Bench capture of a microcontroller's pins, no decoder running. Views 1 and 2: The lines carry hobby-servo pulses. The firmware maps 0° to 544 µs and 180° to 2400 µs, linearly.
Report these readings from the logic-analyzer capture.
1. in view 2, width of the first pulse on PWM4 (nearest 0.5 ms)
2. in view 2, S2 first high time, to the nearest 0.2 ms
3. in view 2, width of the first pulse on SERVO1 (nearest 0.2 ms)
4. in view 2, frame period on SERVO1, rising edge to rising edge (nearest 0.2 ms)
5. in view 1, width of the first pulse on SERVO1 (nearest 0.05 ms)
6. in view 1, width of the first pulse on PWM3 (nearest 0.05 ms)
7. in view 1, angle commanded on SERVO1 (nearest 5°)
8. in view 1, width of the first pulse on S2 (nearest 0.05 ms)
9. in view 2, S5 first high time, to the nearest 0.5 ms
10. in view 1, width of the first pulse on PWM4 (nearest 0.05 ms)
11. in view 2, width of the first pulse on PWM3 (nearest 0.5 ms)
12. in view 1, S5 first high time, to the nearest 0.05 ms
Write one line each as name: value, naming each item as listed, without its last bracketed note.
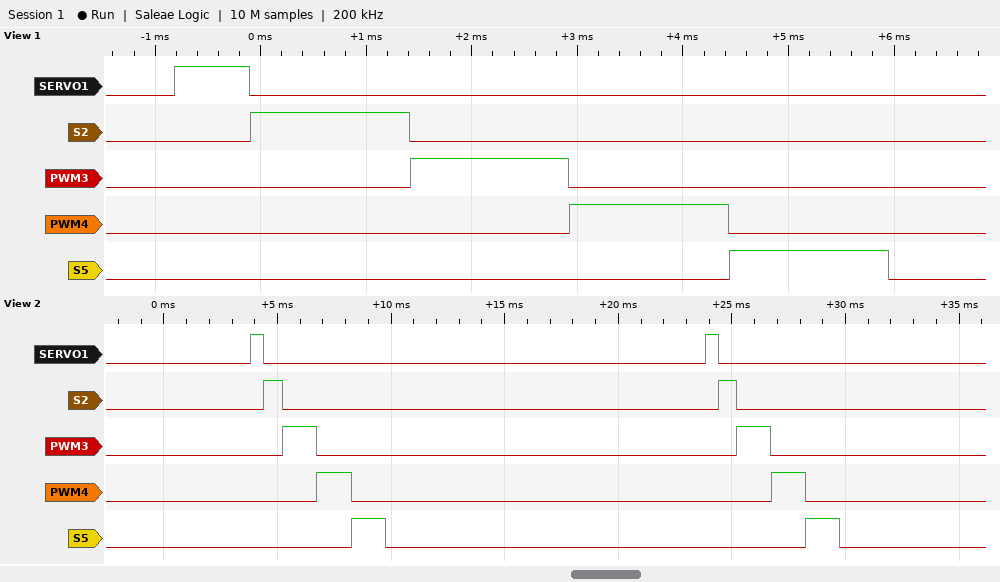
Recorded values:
in view 2, width of the first pulse on PWM4: 1.5 ms
in view 2, S2 first high time, to the nearest 0.2 ms: 0.8 ms
in view 2, width of the first pulse on SERVO1: 0.6 ms
in view 2, frame period on SERVO1, rising edge to rising edge: 20.0 ms
in view 1, width of the first pulse on SERVO1: 0.70 ms
in view 1, width of the first pulse on PWM3: 1.50 ms
in view 1, angle commanded on SERVO1: 15°
in view 1, width of the first pulse on S2: 1.50 ms
in view 2, S5 first high time, to the nearest 0.5 ms: 1.5 ms
in view 1, width of the first pulse on PWM4: 1.50 ms
in view 2, width of the first pulse on PWM3: 1.5 ms
in view 1, S5 first high time, to the nearest 0.05 ms: 1.50 ms
